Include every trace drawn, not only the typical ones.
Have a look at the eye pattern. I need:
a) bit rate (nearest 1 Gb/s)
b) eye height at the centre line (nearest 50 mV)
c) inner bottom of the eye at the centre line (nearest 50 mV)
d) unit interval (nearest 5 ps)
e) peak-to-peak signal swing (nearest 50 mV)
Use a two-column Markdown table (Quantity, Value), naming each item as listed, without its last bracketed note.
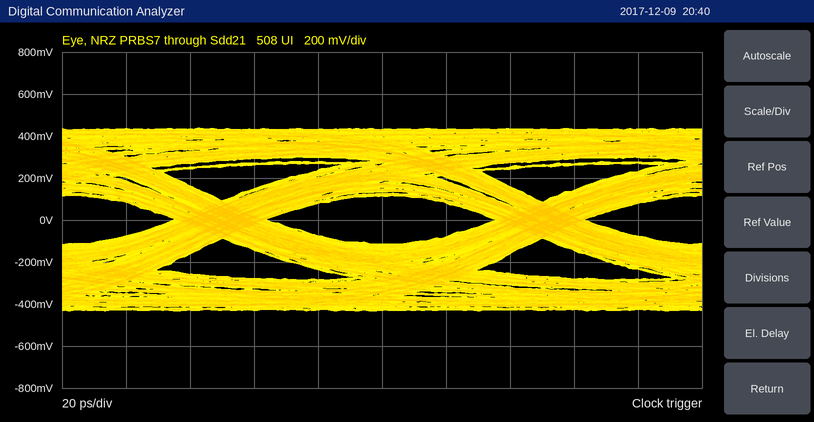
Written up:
| Quantity | Value |
|---|---|
| bit rate | 10 Gb/s |
| eye height at the centre line | 250 mV |
| inner bottom of the eye at the centre line | -100 mV |
| unit interval | 100 ps |
| peak-to-peak signal swing | 850 mV |
